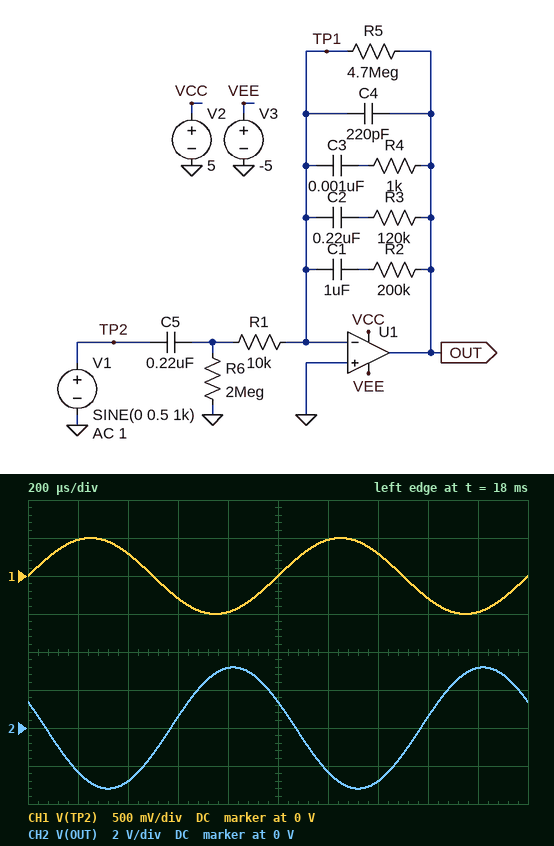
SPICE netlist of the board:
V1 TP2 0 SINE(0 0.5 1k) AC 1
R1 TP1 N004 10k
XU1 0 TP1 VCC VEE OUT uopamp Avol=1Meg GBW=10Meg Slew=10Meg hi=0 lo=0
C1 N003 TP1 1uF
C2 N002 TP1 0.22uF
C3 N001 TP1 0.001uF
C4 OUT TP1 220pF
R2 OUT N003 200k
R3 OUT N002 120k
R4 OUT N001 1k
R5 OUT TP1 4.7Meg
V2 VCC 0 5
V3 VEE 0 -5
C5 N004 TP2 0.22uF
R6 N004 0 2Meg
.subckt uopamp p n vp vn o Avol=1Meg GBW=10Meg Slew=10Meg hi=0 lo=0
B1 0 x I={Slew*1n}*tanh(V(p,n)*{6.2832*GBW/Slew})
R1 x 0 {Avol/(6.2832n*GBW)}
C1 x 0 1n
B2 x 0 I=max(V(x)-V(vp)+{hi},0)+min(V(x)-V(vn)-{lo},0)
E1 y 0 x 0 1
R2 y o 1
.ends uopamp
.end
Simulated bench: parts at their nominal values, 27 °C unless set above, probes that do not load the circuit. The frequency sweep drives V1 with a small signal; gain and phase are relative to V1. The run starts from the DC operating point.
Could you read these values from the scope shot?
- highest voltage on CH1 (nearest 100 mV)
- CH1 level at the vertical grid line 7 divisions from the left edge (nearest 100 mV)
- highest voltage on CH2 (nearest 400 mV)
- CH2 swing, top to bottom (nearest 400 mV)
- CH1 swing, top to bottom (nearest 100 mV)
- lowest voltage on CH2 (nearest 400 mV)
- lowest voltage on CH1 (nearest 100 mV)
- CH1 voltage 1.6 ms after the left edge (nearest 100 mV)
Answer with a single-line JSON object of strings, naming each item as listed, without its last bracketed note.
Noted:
{"highest voltage on CH1": "500 mV", "CH1 level at the vertical grid line 7 divisions from the left edge": "300 mV", "highest voltage on CH2": "3.2 V", "CH2 swing, top to bottom": "6.4 V", "CH1 swing, top to bottom": "1.0 V", "lowest voltage on CH2": "-3.2 V", "lowest voltage on CH1": "-500 mV", "CH1 voltage 1.6 ms after the left edge": "-300 mV"}
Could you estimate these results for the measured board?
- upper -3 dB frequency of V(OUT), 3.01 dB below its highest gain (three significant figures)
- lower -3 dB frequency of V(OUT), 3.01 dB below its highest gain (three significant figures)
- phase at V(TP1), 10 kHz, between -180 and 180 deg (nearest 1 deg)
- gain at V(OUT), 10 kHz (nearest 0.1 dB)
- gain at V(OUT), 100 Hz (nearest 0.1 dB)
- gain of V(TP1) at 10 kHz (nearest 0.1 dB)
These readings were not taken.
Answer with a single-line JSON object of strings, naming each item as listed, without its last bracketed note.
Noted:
{"upper -3 dB frequency of V(OUT), 3.01 dB below its highest gain": "1.89 kHz", "lower -3 dB frequency of V(OUT), 3.01 dB below its highest gain": "66.9 Hz", "phase at V(TP1), 10 kHz, between -180 and 180 deg": "13 deg", "gain at V(OUT), 10 kHz": "2.1 dB", "gain at V(OUT), 100 Hz": "15.5 dB", "gain of V(TP1) at 10 kHz": "-57.9 dB"}
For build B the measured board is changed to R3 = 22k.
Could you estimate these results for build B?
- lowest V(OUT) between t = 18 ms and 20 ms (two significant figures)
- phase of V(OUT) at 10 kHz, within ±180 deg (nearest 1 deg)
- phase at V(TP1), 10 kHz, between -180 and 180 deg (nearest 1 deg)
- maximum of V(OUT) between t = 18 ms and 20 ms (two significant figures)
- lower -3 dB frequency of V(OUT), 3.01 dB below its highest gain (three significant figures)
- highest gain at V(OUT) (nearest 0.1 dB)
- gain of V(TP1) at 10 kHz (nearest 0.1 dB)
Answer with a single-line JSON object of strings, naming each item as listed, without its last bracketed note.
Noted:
{"lowest V(OUT) between t = 18 ms and 20 ms": "-970 mV", "phase of V(OUT) at 10 kHz, within ±180 deg": "126 deg", "phase at V(TP1), 10 kHz, between -180 and 180 deg": "36 deg", "maximum of V(OUT) between t = 18 ms and 20 ms": "970 mV", "lower -3 dB frequency of V(OUT), 3.01 dB below its highest gain": "54.8 Hz", "highest gain at V(OUT)": "5.8 dB", "gain of V(TP1) at 10 kHz": "-59.5 dB"}
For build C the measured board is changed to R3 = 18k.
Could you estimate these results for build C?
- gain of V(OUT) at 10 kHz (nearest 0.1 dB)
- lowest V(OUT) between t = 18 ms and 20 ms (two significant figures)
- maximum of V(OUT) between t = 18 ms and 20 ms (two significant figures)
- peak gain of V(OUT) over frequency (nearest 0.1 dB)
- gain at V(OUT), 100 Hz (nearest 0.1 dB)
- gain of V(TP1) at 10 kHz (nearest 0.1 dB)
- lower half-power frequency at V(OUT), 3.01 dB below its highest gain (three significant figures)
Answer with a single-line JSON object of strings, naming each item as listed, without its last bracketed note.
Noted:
{"gain of V(OUT) at 10 kHz": "0 dB", "lowest V(OUT) between t = 18 ms and 20 ms": "-810 mV", "maximum of V(OUT) between t = 18 ms and 20 ms": "810 mV", "peak gain of V(OUT) over frequency": "4.2 dB", "gain at V(OUT), 100 Hz": "3.1 dB", "gain of V(TP1) at 10 kHz": "-60.0 dB", "lower half-power frequency at V(OUT), 3.01 dB below its highest gain": "44.7 Hz"}
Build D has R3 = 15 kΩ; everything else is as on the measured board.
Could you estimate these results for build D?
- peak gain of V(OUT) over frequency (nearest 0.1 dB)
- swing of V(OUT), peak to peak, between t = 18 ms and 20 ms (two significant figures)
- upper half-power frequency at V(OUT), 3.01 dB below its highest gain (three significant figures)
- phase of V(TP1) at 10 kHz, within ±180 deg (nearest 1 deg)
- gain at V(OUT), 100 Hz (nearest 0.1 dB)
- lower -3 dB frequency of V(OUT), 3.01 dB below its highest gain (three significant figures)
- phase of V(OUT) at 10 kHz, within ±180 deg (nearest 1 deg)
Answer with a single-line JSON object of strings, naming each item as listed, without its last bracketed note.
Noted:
{"peak gain of V(OUT) over frequency": "2.8 dB", "swing of V(OUT), peak to peak, between t = 18 ms and 20 ms": "1.4 V", "upper half-power frequency at V(OUT), 3.01 dB below its highest gain": "9.11 kHz", "phase of V(TP1) at 10 kHz, within ±180 deg": "45 deg", "gain at V(OUT), 100 Hz": "1.9 dB", "lower -3 dB frequency of V(OUT), 3.01 dB below its highest gain": "26.5 Hz", "phase of V(OUT) at 10 kHz, within ±180 deg": "135 deg"}
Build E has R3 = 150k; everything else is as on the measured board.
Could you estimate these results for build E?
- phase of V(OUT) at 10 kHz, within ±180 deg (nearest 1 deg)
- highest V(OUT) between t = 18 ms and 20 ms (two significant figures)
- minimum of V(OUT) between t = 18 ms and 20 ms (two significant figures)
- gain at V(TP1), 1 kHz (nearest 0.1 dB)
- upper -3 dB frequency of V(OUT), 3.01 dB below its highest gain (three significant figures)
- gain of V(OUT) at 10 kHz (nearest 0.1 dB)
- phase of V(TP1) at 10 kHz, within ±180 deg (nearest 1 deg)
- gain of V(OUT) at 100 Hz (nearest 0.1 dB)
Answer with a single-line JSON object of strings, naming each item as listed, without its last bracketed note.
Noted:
{"phase of V(OUT) at 10 kHz, within ±180 deg": "102 deg", "highest V(OUT) between t = 18 ms and 20 ms": "3.5 V", "minimum of V(OUT) between t = 18 ms and 20 ms": "-3.5 V", "gain at V(TP1), 1 kHz": "-63.1 dB", "upper -3 dB frequency of V(OUT), 3.01 dB below its highest gain": "1.68 kHz", "gain of V(OUT) at 10 kHz": "2.1 dB", "phase of V(TP1) at 10 kHz, within ±180 deg": "12 deg", "gain of V(OUT) at 100 Hz": "16.6 dB"}
